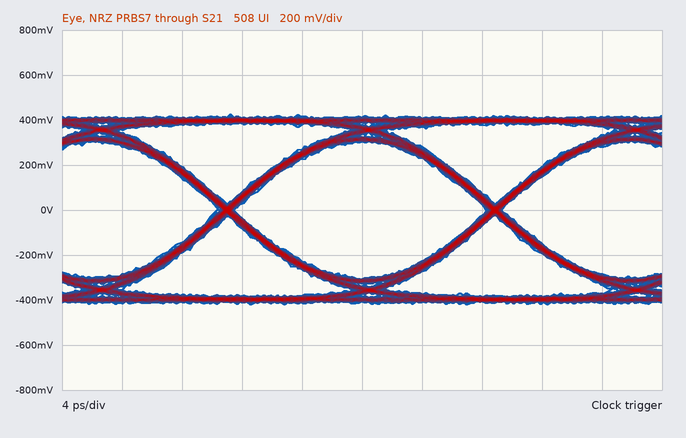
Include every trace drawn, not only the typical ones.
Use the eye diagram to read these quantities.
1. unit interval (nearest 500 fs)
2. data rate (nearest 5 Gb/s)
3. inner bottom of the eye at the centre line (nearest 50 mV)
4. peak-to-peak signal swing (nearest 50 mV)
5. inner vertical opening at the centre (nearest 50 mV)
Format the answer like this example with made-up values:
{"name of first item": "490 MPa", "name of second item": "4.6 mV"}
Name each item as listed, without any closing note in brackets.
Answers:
{"unit interval": "18.0 ps", "data rate": "55 Gb/s", "inner bottom of the eye at the centre line": "-300 mV", "peak-to-peak signal swing": "850 mV", "inner vertical opening at the centre": "600 mV"}
